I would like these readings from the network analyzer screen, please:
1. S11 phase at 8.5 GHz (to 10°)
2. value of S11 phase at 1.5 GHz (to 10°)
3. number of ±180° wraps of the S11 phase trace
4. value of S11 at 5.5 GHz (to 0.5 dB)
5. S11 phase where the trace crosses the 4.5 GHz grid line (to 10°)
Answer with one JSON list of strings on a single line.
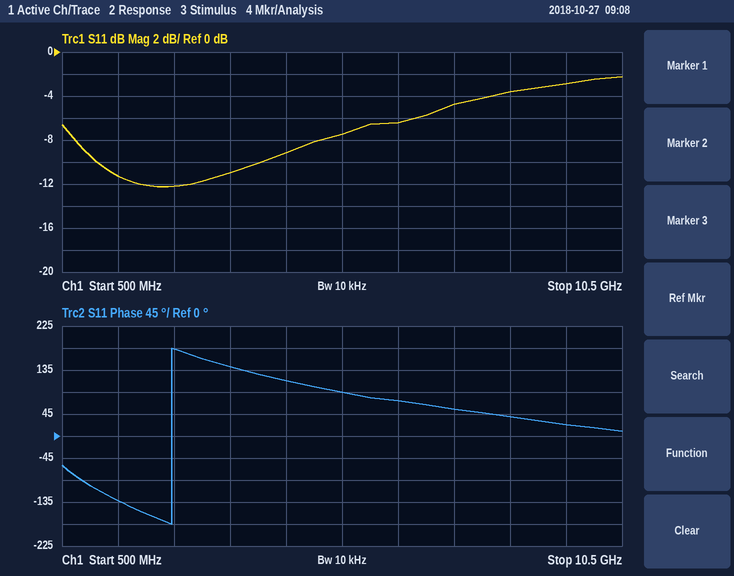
["40°", "-130°", "1", "-7.5 dB", "110°"]
